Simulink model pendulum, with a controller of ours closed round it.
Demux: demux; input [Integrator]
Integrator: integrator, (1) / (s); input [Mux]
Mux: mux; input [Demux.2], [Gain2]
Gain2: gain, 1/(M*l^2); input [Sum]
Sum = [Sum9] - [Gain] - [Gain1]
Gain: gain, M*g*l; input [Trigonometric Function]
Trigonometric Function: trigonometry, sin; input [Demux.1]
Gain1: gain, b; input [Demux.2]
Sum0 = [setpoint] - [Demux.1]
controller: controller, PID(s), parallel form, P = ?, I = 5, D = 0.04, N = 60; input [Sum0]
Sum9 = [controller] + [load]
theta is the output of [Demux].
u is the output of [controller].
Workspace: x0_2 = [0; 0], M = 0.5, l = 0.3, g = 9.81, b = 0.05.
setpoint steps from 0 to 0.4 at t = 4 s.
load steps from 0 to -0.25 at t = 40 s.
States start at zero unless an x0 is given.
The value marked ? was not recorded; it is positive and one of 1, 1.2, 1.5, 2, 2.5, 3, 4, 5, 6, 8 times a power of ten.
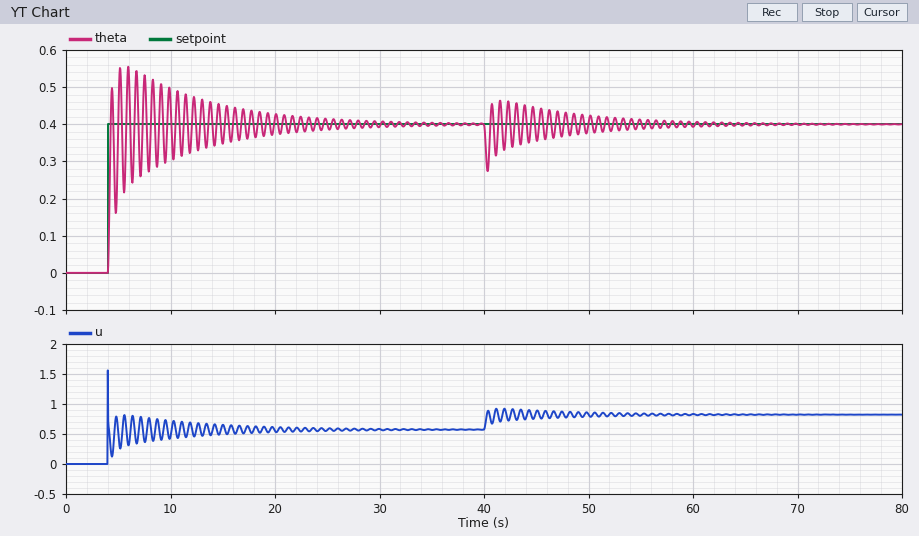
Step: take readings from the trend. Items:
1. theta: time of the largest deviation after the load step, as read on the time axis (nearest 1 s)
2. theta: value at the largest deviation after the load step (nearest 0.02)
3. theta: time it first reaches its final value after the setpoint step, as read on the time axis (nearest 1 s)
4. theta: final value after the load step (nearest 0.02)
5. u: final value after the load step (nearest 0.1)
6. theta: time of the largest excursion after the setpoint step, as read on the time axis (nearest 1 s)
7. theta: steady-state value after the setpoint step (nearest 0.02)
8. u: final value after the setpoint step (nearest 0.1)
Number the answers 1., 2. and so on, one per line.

1. 40 s
2. 0.28
3. 4 s
4. 0.40
5. 0.8
6. 6 s
7. 0.40
8. 0.6
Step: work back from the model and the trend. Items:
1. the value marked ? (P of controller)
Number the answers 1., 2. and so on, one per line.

1. 1.5
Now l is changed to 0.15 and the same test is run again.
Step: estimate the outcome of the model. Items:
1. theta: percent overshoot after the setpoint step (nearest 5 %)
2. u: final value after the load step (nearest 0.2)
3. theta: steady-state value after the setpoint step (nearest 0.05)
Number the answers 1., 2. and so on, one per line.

1. 20 %
2. 0.6
3. 0.40
